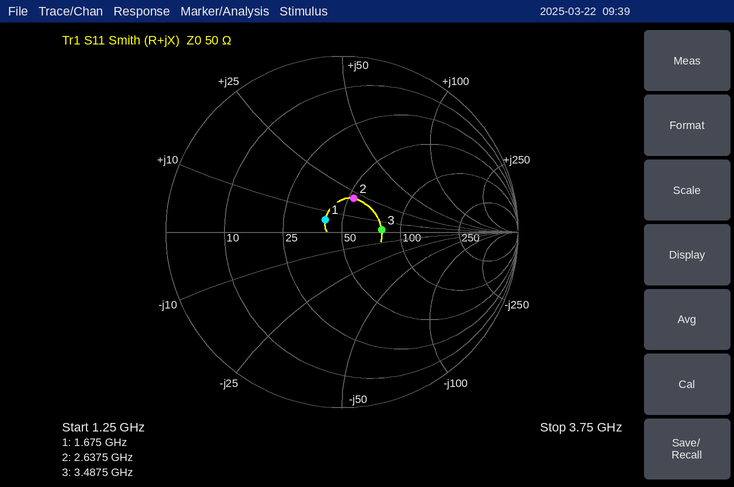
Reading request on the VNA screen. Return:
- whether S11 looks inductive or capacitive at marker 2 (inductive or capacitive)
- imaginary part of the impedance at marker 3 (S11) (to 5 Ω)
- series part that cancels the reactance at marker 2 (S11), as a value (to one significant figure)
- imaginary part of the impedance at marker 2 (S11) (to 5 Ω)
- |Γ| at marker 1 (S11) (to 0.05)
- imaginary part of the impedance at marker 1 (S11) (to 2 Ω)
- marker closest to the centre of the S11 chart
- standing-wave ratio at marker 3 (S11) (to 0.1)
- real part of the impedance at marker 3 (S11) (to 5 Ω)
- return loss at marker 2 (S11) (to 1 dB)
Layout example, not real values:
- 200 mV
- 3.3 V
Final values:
- inductive
- 0 Ω
- 3 pF
- +20 Ω
- 0.10
- +6 Ω
- marker 1
- 1.6
- 80 Ω
- 14 dB
